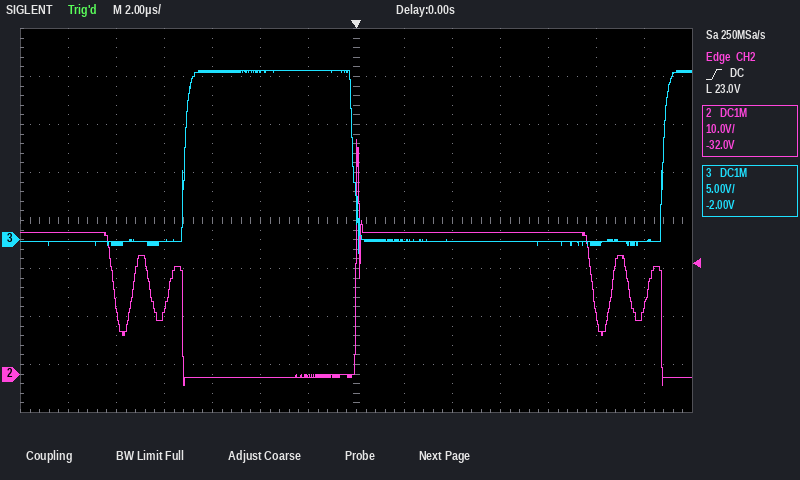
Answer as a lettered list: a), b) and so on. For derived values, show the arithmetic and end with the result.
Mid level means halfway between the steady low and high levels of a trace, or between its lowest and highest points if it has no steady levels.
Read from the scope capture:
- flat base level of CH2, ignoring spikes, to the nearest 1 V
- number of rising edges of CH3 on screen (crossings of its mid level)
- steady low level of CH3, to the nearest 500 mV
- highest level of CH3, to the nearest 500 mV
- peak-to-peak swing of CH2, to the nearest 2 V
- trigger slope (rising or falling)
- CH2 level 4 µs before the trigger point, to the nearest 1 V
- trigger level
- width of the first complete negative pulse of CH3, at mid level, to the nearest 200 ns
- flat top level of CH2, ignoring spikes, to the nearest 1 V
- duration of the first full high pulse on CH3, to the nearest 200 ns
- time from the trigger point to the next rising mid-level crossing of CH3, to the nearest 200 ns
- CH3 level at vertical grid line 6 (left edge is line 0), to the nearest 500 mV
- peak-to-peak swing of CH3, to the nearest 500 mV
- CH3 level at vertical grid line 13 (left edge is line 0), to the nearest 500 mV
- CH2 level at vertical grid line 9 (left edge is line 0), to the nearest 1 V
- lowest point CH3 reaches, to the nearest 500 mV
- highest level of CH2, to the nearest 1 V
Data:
a) -1 V
b) 2
c) 0.0 V
d) 17.5 V
e) 52 V
f) rising
g) -1 V
h) 23.0 V
i) 13.0 µs
j) 30 V
k) 7.0 µs
l) 12.8 µs
m) 17.5 V
n) 17.5 V − (-1.5 V) = 19.0 V
o) 0.0 V
p) 30 V
q) -1.5 V
r) 49 V
